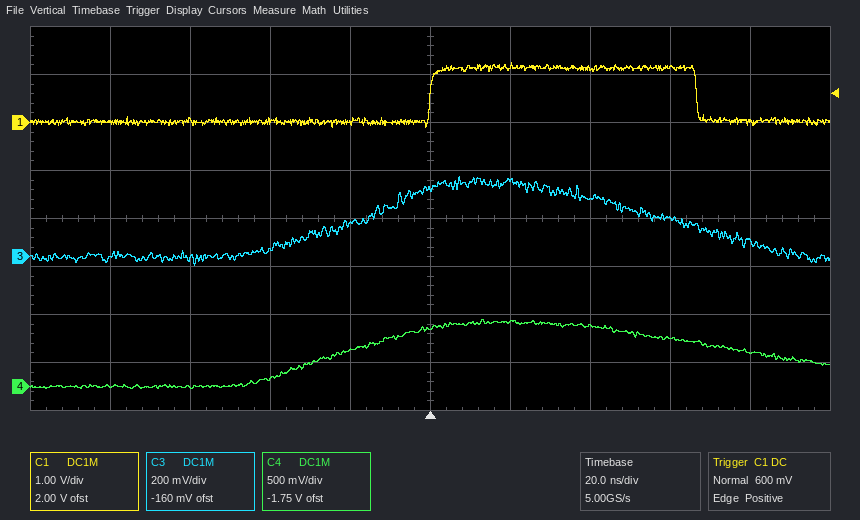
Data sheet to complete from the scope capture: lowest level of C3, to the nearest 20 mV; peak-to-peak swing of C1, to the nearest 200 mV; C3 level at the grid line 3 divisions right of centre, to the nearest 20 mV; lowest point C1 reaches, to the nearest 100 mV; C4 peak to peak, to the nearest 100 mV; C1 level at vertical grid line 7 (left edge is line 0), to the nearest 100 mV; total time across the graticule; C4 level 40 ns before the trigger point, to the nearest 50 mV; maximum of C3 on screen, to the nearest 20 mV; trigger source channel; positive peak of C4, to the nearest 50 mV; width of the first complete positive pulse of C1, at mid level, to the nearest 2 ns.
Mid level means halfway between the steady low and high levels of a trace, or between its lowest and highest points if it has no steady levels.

-40 mV
1.4 V
160 mV
-100 mV
700 mV
1.1 V
200 ns
100 mV
340 mV
C1
700 mV
66 ns
